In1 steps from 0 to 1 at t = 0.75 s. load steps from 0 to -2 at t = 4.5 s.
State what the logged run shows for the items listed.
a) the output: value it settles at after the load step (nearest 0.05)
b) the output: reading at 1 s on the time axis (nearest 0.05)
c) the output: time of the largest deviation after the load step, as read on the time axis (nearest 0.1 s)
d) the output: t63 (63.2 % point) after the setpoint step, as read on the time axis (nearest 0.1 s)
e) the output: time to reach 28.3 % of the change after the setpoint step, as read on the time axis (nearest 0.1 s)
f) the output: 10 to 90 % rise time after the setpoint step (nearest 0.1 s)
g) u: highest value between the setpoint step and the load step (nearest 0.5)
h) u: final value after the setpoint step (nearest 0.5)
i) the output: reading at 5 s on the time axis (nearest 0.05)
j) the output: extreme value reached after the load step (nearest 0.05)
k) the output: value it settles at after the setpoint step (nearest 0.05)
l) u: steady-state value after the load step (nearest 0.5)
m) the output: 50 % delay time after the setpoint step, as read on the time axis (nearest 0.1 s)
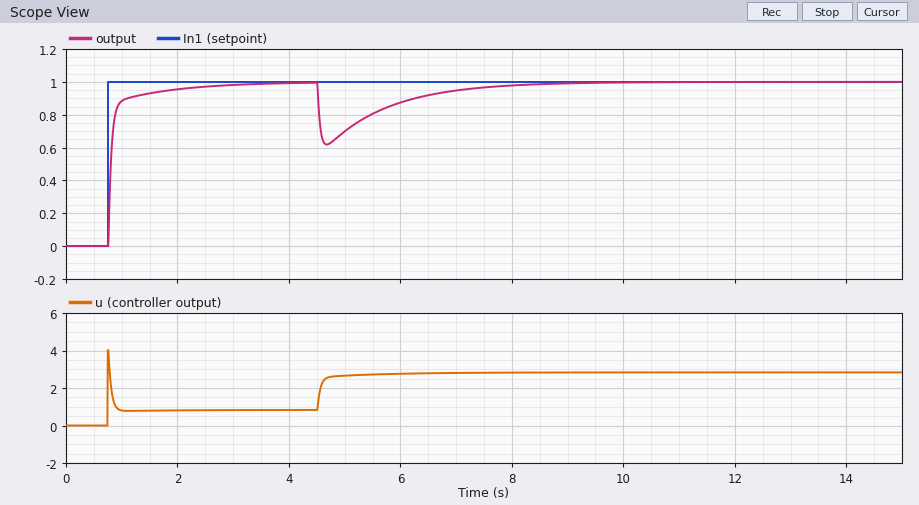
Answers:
1.00
0.90
4.7 s
0.8 s
0.8 s
0.3 s
4.0
1.0
0.70
0.60
1.00
3.0
0.8 s
